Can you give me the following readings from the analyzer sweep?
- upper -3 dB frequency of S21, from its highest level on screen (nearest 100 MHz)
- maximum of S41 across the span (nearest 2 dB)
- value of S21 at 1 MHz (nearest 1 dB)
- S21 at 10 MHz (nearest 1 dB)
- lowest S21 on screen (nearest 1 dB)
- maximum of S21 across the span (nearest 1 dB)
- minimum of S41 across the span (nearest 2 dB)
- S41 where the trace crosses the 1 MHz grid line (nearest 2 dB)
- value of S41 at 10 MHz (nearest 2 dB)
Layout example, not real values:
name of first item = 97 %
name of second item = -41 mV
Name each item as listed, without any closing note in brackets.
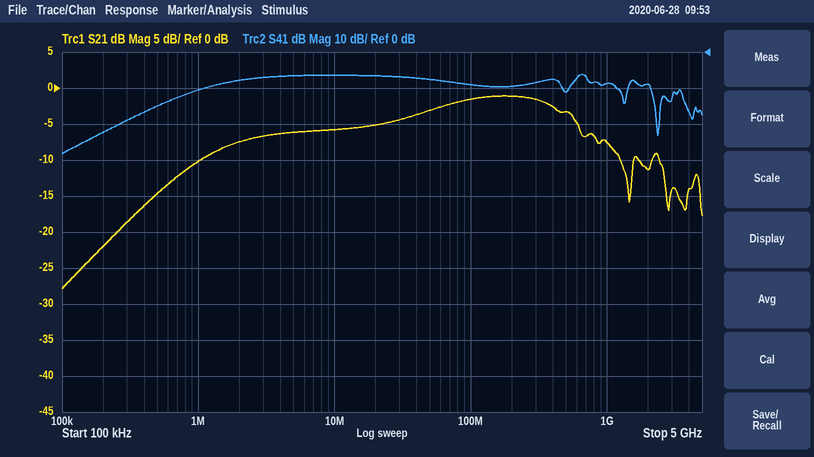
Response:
upper -3 dB frequency of S21, from its highest level on screen = 600 MHz
maximum of S41 across the span = -6 dB
value of S21 at 1 MHz = -10 dB
S21 at 10 MHz = -6 dB
lowest S21 on screen = -28 dB
maximum of S21 across the span = -1 dB
minimum of S41 across the span = -28 dB
S41 where the trace crosses the 1 MHz grid line = -10 dB
value of S41 at 10 MHz = -6 dB
